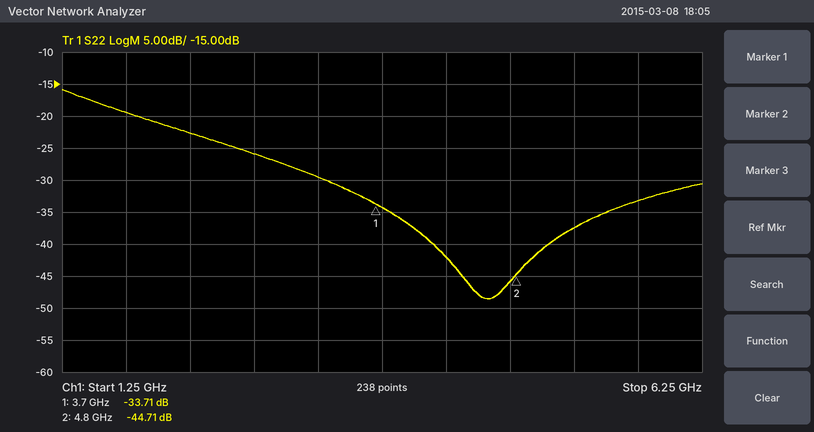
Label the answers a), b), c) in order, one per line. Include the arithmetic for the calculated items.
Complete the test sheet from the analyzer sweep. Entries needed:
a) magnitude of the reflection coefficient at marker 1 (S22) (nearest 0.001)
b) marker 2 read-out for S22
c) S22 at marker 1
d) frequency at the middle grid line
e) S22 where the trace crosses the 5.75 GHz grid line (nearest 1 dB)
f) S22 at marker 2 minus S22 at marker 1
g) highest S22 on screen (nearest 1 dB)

a) 10^(-33.71/20) ≈ 0.021
b) -44.71 dB
c) -33.71 dB
d) 3.75 GHz
e) -33 dB
f) -44.71 − (-33.71) = -11.00 dB
g) -16 dB
